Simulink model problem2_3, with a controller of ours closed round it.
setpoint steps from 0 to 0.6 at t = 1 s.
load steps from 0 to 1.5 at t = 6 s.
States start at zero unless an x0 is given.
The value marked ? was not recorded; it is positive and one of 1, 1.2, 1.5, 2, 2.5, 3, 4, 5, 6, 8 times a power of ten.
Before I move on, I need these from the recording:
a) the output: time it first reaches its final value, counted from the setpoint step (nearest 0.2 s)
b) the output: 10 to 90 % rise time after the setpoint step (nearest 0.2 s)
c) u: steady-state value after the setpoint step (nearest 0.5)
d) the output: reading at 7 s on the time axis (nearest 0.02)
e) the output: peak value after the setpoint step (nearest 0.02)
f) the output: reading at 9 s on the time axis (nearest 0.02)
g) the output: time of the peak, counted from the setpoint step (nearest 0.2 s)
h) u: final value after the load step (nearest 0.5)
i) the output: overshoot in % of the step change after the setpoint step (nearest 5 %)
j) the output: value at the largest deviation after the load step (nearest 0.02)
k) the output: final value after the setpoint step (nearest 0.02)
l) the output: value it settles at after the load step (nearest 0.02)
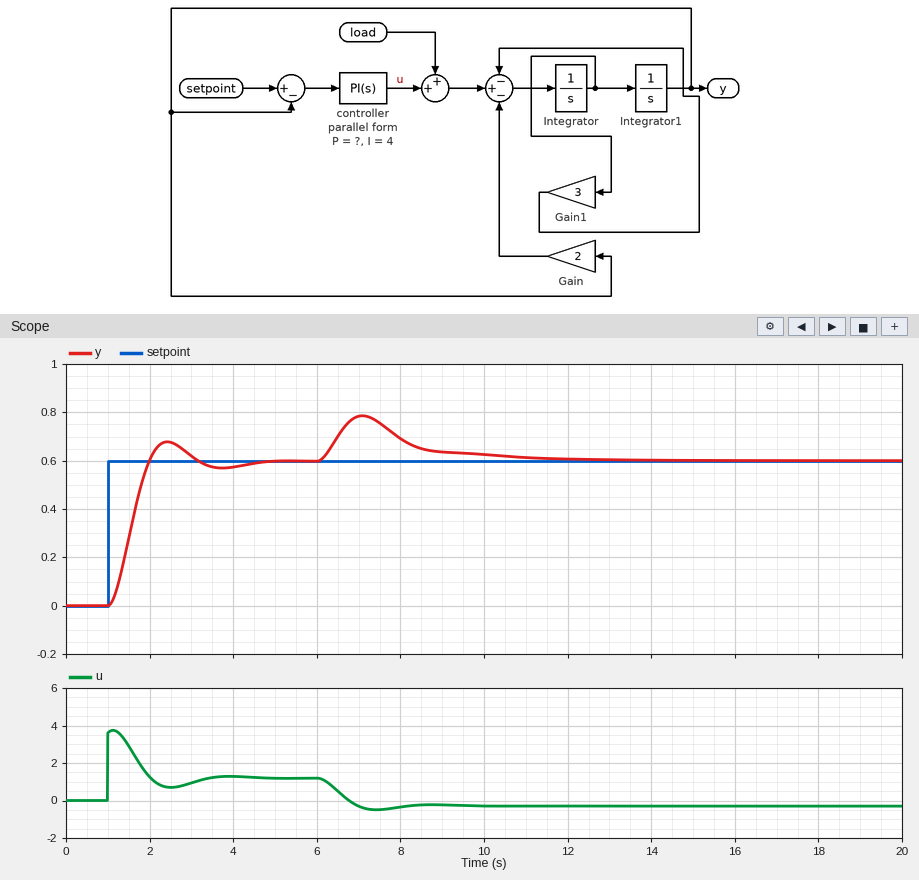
1.0 s
0.6 s
1.0
0.78
0.68
0.64
1.4 s
-0.5
15 %
0.78
0.60
0.60
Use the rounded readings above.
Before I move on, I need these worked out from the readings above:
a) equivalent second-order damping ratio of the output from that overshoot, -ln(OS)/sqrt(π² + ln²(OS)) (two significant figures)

0.52
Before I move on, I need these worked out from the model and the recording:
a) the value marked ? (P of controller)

6
